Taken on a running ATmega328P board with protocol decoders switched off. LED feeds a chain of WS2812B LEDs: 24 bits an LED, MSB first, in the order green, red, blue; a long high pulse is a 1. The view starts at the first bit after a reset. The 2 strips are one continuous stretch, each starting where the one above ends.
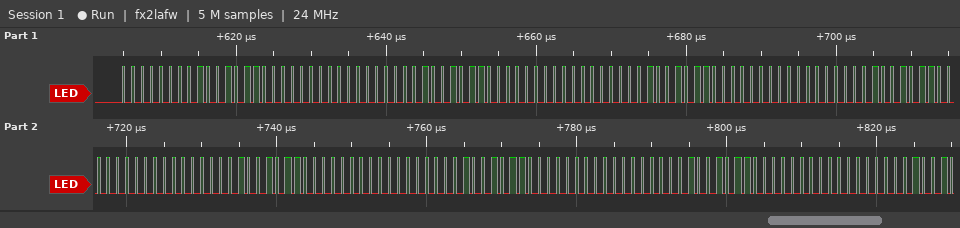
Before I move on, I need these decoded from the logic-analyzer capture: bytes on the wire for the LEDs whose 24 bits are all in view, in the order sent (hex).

00 96 00 00 96 00 00 96 00 00 96 00 00 96 00 00 96 00 00 96 00
